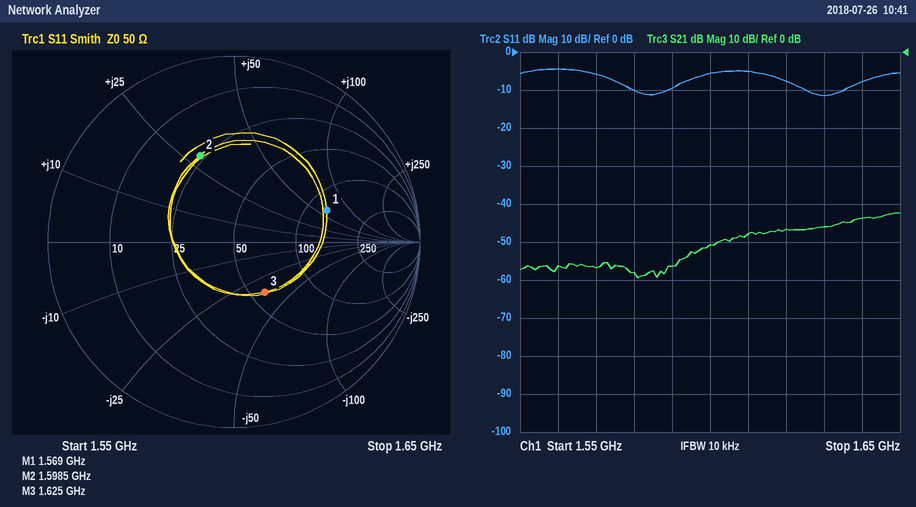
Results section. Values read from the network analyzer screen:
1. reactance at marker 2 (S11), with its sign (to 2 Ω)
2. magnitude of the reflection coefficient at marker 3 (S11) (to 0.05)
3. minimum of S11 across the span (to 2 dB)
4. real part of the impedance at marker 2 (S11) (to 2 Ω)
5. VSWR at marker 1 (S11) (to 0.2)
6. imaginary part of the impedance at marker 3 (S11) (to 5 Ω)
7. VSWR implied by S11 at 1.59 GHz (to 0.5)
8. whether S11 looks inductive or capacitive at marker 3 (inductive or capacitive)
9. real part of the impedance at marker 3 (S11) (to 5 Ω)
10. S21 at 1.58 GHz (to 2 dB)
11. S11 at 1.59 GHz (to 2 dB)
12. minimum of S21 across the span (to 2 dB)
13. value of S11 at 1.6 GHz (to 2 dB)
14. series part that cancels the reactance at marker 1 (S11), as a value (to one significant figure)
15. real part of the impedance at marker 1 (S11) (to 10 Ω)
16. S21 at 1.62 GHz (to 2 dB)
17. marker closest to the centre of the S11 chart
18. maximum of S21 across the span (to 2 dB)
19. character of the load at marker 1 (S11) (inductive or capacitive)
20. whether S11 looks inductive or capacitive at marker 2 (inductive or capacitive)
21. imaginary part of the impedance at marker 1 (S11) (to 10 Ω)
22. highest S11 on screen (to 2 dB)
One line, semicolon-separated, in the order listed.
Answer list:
+28 Ω; 0.30; -12 dB; 24 Ω; 3.2; -35 Ω; 2.0; capacitive; 60 Ω; -58 dB; -10 dB; -60 dB; -6 dB; 2 pF; 130 Ω; -46 dB; marker 3; -42 dB; inductive; inductive; +60 Ω; -4 dB
